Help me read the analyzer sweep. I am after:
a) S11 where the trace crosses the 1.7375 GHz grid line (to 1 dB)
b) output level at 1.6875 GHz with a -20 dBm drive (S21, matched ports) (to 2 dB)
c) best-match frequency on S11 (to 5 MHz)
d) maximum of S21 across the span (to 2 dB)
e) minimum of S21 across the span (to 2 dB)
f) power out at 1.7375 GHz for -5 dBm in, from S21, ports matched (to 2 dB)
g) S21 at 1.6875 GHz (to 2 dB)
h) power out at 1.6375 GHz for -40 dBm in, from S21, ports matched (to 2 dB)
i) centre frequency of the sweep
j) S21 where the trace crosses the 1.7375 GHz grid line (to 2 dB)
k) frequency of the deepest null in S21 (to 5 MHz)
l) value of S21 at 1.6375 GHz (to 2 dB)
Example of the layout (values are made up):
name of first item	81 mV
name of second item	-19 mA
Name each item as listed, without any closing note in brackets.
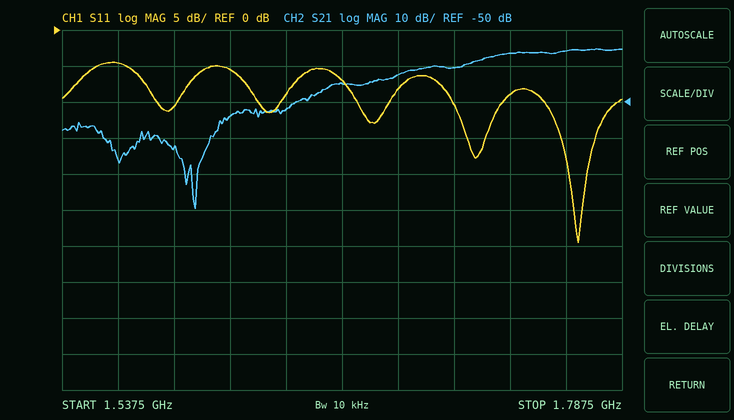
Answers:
S11 where the trace crosses the 1.7375 GHz grid line	-9 dB
output level at 1.6875 GHz with a -20 dBm drive (S21, matched ports)	-62 dBm
best-match frequency on S11	1.770 GHz
maximum of S21 across the span	-36 dB
minimum of S21 across the span	-80 dB
power out at 1.7375 GHz for -5 dBm in, from S21, ports matched	-42 dBm
S21 at 1.6875 GHz	-42 dB
power out at 1.6375 GHz for -40 dBm in, from S21, ports matched	-92 dBm
centre frequency of the sweep	1.6625 GHz
S21 where the trace crosses the 1.7375 GHz grid line	-36 dB
frequency of the deepest null in S21	1.595 GHz
value of S21 at 1.6375 GHz	-52 dB
